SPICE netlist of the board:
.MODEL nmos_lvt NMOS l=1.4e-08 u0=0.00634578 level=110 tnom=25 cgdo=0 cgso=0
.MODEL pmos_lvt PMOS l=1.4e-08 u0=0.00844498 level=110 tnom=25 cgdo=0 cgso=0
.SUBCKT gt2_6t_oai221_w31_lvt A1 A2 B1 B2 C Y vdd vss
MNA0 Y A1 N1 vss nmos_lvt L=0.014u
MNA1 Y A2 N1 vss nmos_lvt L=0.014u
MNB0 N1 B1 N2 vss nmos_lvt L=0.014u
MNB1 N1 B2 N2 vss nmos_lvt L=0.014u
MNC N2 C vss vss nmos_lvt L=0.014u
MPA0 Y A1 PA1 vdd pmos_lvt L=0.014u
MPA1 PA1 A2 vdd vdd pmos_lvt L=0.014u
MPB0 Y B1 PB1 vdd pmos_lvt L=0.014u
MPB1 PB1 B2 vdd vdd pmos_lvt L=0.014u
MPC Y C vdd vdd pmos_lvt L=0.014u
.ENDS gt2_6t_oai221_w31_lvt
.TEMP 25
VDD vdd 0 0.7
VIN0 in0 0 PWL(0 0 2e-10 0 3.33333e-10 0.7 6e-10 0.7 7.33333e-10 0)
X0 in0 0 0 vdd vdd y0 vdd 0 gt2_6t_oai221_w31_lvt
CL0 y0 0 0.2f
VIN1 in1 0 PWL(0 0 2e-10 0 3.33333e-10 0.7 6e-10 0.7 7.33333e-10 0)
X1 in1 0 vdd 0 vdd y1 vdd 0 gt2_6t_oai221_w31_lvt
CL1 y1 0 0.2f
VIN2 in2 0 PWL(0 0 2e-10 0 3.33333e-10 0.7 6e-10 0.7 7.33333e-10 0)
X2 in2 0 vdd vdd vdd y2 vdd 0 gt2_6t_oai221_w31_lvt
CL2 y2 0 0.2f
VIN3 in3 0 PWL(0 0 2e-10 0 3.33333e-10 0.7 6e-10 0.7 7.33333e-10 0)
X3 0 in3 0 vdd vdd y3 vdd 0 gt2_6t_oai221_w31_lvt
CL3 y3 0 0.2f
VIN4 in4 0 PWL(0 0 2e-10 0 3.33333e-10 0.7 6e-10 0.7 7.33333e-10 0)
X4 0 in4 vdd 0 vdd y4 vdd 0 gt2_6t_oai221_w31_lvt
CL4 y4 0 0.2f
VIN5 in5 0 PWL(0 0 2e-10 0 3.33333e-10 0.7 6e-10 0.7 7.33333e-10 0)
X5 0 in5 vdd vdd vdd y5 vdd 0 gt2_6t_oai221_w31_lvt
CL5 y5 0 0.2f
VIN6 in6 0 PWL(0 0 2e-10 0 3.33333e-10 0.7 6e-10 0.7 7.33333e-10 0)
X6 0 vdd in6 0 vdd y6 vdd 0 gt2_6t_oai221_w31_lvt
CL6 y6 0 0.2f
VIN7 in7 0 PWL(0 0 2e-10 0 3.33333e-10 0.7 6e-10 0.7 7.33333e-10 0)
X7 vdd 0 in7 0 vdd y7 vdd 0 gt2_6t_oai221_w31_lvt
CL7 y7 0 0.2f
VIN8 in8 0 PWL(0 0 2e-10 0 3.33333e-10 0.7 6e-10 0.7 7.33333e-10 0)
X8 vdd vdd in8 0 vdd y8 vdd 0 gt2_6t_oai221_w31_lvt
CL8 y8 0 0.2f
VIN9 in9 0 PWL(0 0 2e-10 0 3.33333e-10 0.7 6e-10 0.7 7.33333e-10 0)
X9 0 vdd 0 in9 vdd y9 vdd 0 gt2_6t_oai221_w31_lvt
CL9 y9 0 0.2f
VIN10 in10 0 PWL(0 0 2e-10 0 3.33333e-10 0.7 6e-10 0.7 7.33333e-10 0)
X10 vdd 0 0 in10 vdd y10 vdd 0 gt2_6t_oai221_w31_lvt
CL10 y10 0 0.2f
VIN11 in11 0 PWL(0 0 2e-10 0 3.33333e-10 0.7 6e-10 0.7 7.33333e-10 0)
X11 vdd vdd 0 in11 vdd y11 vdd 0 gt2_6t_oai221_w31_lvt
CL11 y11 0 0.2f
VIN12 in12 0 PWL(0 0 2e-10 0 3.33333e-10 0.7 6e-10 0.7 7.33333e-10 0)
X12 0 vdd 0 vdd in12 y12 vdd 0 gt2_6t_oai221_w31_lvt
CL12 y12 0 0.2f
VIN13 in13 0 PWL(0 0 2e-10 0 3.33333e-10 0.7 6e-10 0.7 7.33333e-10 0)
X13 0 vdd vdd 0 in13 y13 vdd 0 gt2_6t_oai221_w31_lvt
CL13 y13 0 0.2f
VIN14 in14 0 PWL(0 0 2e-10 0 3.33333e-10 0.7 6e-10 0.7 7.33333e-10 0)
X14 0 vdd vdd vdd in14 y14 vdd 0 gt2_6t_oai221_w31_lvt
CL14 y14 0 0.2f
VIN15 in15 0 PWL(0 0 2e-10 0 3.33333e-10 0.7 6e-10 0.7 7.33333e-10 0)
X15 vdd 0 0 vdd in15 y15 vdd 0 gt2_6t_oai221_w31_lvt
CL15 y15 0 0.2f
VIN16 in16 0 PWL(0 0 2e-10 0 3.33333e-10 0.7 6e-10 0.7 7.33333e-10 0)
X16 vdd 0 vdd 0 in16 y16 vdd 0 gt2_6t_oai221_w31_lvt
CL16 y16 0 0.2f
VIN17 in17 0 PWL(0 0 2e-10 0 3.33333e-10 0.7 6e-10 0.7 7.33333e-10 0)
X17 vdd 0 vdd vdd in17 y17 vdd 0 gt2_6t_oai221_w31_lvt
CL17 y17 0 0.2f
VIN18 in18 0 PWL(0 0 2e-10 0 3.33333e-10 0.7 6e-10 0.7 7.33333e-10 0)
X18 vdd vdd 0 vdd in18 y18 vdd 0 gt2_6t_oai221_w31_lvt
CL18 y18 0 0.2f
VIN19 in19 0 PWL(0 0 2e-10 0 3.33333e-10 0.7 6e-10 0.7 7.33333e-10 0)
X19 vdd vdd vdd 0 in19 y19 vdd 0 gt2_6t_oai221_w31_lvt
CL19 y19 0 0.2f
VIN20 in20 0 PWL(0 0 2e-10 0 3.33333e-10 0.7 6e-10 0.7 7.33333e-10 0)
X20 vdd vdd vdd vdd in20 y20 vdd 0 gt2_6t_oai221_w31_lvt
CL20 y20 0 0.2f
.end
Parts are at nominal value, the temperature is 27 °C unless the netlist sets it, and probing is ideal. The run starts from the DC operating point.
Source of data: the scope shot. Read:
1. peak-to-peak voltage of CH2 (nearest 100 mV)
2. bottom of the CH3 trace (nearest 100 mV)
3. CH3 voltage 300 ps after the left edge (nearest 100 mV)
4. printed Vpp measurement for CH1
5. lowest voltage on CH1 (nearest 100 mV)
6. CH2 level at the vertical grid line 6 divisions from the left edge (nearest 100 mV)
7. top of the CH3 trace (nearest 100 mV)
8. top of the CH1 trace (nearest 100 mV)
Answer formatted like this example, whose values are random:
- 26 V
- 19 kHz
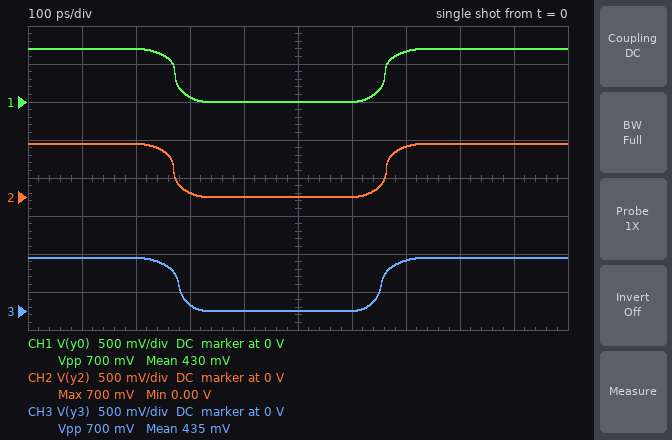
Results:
- 700 mV
- 0 V
- 100 mV
- 700 mV
- 0 V
- 0 V
- 700 mV
- 700 mV
